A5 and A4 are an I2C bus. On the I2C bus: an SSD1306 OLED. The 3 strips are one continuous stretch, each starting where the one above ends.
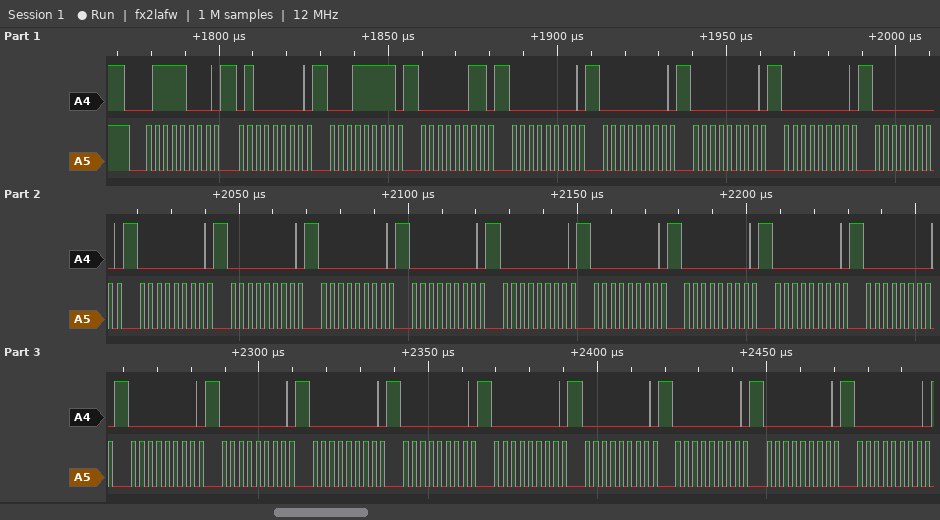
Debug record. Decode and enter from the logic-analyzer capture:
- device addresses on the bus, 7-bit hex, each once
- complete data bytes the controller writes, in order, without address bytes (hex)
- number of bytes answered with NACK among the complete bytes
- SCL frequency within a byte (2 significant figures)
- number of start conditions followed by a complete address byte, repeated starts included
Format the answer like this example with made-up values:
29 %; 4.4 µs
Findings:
0x3C; 40 1F 03 00 00 00 00 00 00 00 00 00 00 00 00 00 00 00 00 00 00 00 00 00 00 00; 0; 400 kHz; 1
